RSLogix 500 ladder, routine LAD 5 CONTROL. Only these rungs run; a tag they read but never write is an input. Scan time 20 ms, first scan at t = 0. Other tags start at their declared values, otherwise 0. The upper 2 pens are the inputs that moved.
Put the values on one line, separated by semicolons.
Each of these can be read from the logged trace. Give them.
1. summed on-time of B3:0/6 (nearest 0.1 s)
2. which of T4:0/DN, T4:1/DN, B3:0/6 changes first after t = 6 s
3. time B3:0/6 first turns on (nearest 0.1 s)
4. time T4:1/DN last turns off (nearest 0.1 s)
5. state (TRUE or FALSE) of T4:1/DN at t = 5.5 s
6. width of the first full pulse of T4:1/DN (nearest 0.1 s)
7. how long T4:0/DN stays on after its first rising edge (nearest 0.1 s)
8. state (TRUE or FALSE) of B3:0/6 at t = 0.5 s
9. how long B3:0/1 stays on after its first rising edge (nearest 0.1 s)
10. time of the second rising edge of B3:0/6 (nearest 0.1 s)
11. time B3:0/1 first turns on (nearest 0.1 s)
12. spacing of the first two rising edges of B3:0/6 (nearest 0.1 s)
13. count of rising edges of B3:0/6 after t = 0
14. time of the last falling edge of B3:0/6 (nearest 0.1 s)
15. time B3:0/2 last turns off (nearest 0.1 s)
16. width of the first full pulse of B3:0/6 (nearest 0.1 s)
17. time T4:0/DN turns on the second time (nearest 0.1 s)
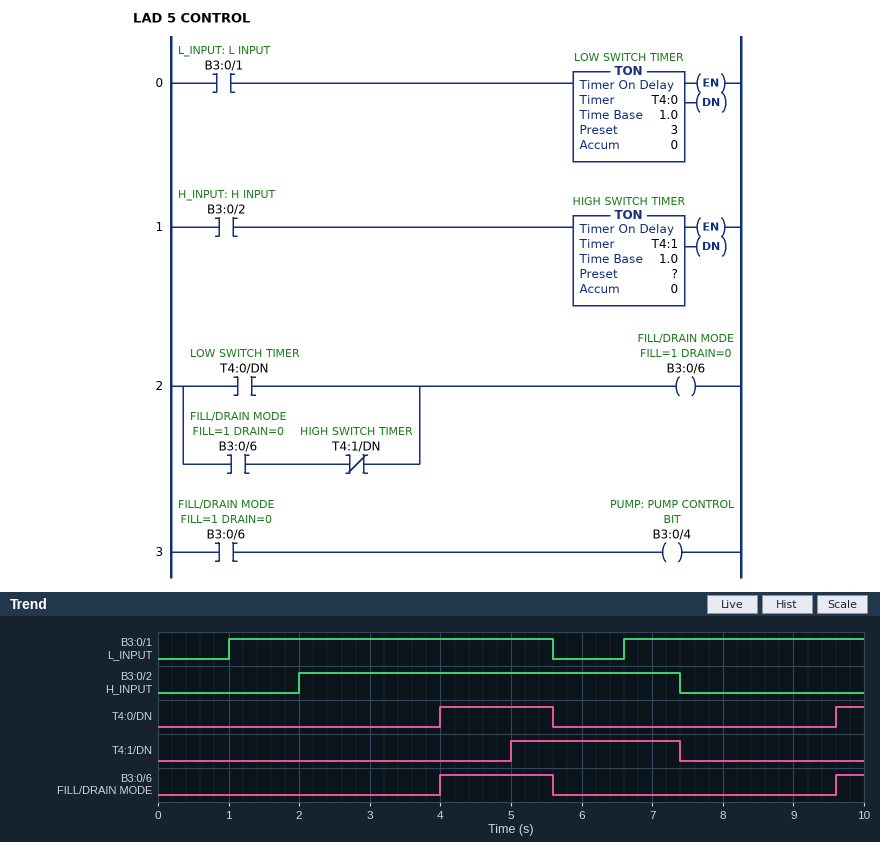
2.0 s; T4:1/DN; 4.0 s; 7.4 s; TRUE; 2.4 s; 1.6 s; FALSE; 4.6 s; 9.6 s; 1.0 s; 5.6 s; 2; 5.6 s; 7.4 s; 1.6 s; 9.6 s
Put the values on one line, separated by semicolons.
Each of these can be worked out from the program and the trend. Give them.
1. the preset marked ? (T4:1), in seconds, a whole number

3 s
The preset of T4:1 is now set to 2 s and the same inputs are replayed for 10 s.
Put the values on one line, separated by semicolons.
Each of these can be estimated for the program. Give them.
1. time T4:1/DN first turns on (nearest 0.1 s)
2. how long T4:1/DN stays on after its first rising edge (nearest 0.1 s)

4.0 s; 3.4 s
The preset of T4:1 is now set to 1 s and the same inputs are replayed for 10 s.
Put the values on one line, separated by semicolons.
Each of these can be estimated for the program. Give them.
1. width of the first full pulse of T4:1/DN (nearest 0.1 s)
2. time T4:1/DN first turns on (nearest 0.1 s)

4.4 s; 3.0 s
